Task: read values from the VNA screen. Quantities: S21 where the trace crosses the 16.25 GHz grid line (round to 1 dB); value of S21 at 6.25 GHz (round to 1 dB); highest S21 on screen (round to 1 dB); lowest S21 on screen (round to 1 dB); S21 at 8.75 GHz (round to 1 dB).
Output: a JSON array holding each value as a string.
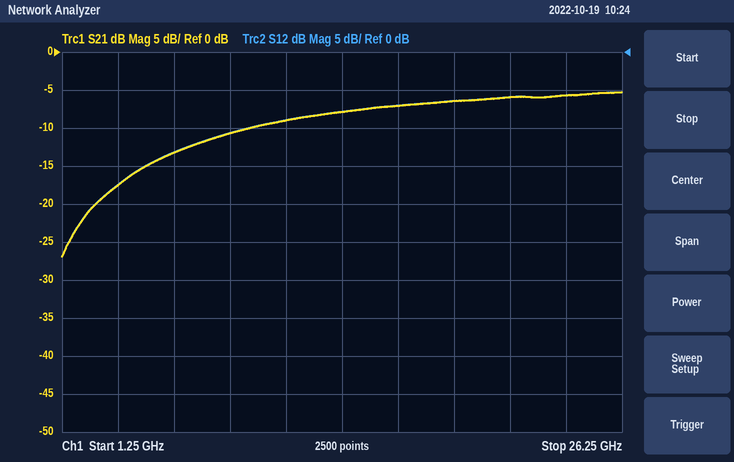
["-7 dB", "-13 dB", "-5 dB", "-27 dB", "-11 dB"]
